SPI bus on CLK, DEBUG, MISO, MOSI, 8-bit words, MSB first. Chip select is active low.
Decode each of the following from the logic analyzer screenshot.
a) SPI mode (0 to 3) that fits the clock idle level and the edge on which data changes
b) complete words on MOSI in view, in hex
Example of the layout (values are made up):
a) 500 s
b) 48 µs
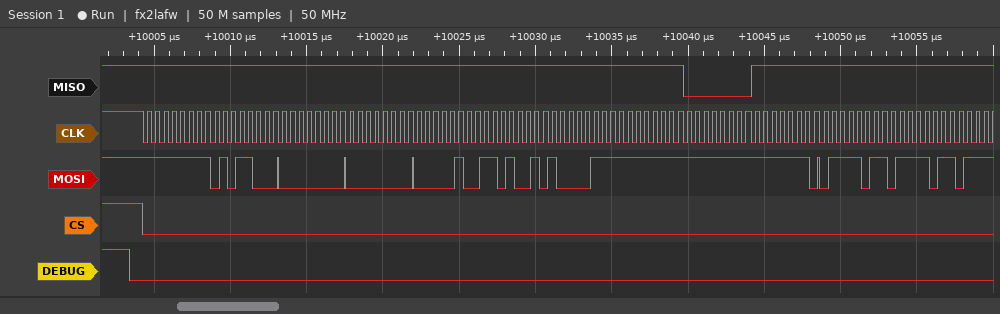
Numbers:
a) 3
b) FF, 58, 00, 00, 04, D2, 87, FF, FF, FE, 7B, 7B
